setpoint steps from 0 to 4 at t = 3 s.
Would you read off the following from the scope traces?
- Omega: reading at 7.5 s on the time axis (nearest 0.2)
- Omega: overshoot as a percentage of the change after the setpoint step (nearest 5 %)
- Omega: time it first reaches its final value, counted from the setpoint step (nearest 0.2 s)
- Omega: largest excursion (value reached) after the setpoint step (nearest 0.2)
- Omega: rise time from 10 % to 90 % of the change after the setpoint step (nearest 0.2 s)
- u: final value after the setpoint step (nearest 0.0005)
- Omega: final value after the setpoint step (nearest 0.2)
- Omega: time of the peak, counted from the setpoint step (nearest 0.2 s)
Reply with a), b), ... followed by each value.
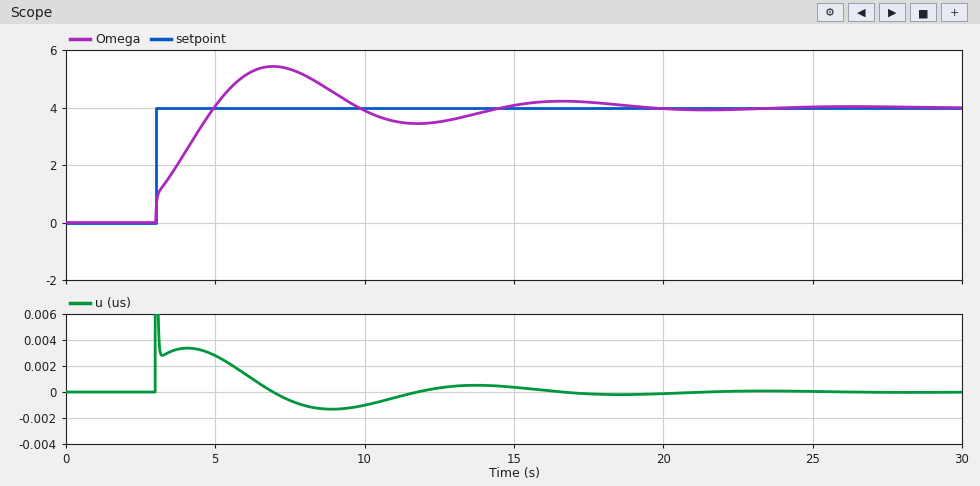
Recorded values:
a) 5.4
b) 35 %
c) 2.0 s
d) 5.4
e) 1.6 s
f) 0.0000
g) 4.0
h) 4.0 s
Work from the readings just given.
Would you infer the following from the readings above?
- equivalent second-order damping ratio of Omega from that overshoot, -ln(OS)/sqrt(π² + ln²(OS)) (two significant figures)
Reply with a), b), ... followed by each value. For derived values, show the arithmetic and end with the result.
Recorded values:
a) ln(0.35) = -1.050; 1.050 / sqrt(9.870 + 1.102) = 0.32
